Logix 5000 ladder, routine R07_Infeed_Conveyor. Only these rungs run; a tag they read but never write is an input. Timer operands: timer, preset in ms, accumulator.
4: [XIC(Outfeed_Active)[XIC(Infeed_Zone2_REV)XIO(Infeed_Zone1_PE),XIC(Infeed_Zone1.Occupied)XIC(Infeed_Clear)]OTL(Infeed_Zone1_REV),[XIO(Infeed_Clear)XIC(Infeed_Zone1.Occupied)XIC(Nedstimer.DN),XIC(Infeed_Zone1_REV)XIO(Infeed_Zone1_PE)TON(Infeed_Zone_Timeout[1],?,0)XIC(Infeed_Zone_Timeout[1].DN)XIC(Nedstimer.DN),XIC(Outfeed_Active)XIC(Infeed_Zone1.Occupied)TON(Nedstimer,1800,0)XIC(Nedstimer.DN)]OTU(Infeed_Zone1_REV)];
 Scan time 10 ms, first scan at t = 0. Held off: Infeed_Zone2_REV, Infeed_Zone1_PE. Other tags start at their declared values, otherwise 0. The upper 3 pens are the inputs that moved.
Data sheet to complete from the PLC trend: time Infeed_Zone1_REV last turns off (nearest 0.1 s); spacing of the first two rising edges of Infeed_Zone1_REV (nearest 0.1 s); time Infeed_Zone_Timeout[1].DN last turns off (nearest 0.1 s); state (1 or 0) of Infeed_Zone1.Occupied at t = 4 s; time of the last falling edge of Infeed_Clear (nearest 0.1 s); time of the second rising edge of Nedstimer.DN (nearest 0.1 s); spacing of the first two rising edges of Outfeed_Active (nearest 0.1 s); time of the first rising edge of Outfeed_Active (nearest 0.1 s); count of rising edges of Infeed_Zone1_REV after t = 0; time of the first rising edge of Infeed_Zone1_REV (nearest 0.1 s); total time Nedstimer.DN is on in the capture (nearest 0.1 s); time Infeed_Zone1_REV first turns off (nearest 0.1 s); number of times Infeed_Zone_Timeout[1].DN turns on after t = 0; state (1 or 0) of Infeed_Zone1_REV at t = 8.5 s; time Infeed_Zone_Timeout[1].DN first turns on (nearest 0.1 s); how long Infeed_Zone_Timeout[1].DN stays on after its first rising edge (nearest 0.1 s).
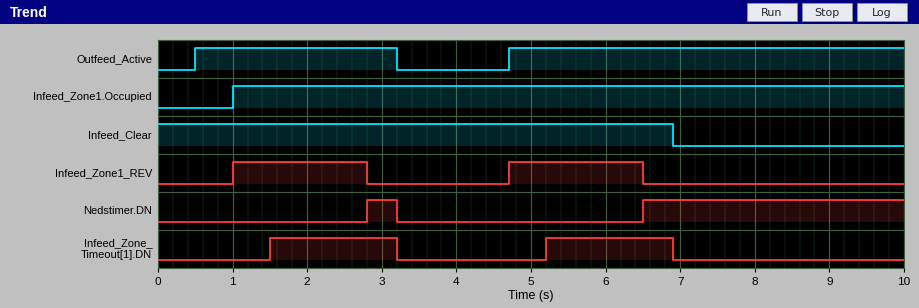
6.5 s
3.7 s
6.9 s
1
6.9 s
6.5 s
4.2 s
0.5 s
2
1.0 s
3.9 s
2.8 s
2
0
1.5 s
1.7 s
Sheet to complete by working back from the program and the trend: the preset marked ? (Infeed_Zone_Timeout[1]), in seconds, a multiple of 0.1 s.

0.5 s
